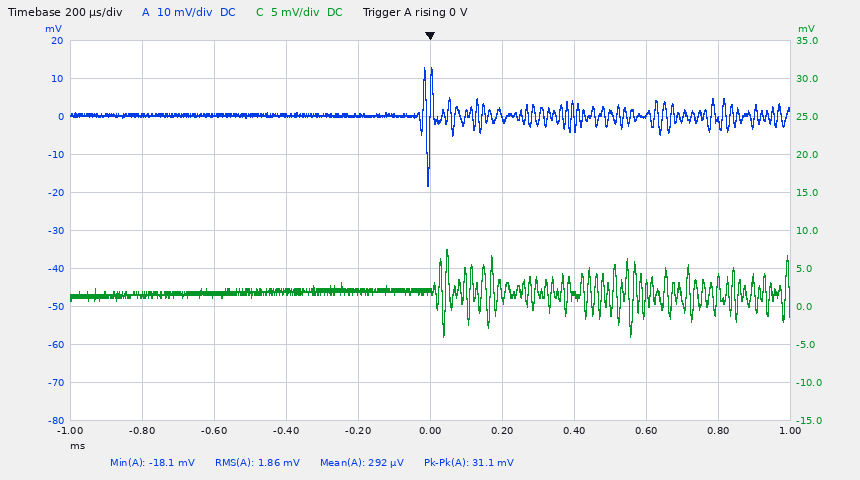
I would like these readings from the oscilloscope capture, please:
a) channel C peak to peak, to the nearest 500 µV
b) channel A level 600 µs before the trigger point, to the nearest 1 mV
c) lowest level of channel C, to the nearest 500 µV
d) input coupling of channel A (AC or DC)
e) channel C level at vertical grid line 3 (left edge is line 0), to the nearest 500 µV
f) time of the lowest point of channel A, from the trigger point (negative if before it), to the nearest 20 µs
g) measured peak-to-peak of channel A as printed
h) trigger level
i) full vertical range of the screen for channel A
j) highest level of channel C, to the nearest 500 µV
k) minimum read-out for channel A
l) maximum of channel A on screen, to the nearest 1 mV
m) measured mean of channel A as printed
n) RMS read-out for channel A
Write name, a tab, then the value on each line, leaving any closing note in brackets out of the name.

channel C peak to peak, to the nearest 500 µV	11.5 mV
channel A level 600 µs before the trigger point, to the nearest 1 mV	0 mV
lowest level of channel C, to the nearest 500 µV	-4.0 mV
input coupling of channel A	DC
channel C level at vertical grid line 3 (left edge is line 0), to the nearest 500 µV	2.0 mV
time of the lowest point of channel A, from the trigger point (negative if before it), to the nearest 20 µs	0 µs
measured peak-to-peak of channel A as printed	31.1 mV
trigger level	0 V
full vertical range of the screen for channel A	100 mV
highest level of channel C, to the nearest 500 µV	7.5 mV
minimum read-out for channel A	-18.1 mV
maximum of channel A on screen, to the nearest 1 mV	13 mV
measured mean of channel A as printed	292 µV
RMS read-out for channel A	1.86 mV
